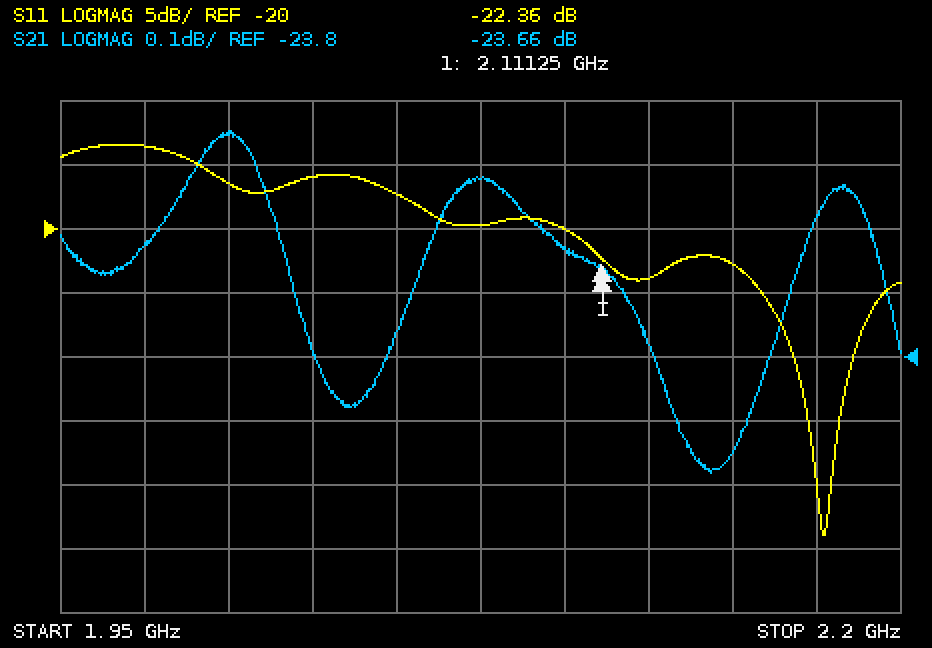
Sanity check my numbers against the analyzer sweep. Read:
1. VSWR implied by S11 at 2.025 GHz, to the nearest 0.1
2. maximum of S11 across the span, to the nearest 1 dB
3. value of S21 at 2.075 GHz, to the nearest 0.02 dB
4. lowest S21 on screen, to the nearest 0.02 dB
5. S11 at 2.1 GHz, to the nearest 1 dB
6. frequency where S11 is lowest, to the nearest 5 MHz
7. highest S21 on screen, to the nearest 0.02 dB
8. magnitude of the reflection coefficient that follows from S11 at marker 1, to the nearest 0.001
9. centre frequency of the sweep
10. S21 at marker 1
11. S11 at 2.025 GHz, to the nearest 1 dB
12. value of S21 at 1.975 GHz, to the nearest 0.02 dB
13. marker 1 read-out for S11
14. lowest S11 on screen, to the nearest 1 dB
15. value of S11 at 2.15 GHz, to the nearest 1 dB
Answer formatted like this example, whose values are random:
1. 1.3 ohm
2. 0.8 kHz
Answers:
1. 1.4
2. -13 dB
3. -23.52 dB
4. -23.98 dB
5. -20 dB
6. 2.175 GHz
7. -23.44 dB
8. 0.076
9. 2.075 GHz
10. -23.66 dB
11. -16 dB
12. -23.62 dB
13. -22.36 dB
14. -44 dB
15. -23 dB
